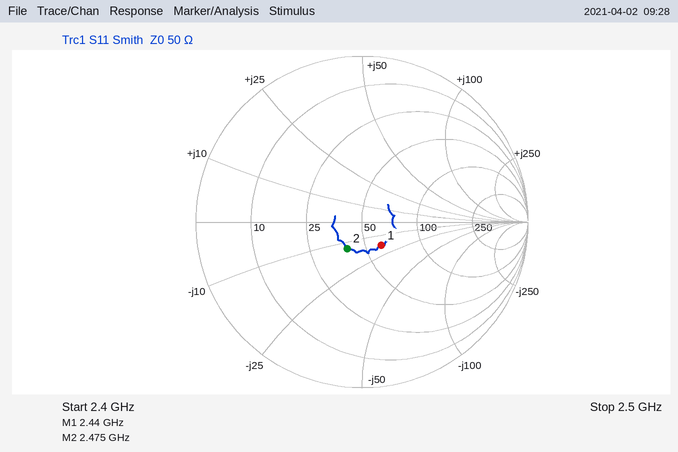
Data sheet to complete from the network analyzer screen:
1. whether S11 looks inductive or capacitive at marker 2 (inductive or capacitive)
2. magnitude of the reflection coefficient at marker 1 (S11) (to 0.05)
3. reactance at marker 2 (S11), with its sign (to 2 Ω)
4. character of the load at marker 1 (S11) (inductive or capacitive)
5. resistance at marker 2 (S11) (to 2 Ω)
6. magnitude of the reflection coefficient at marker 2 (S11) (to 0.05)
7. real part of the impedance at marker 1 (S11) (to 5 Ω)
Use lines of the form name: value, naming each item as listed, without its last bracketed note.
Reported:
whether S11 looks inductive or capacitive at marker 2: capacitive
magnitude of the reflection coefficient at marker 1 (S11): 0.20
reactance at marker 2 (S11), with its sign: -14 Ω
character of the load at marker 1 (S11): capacitive
resistance at marker 2 (S11): 40 Ω
magnitude of the reflection coefficient at marker 2 (S11): 0.20
real part of the impedance at marker 1 (S11): 60 Ω
